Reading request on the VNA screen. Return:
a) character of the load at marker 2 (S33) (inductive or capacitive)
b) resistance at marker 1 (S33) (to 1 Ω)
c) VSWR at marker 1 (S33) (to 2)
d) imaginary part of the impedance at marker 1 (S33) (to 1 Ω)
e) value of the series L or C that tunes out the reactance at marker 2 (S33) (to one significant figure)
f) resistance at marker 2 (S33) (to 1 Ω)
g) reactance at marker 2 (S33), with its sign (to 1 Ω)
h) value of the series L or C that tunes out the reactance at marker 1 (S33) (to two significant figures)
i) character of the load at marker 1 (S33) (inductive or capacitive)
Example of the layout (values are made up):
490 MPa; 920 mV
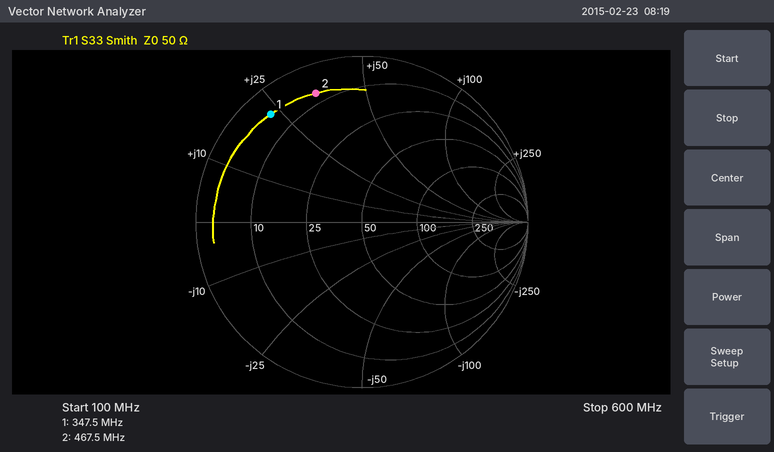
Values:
inductive; 5 Ω; 12; +23 Ω; 10 pF; 7 Ω; +35 Ω; 20 pF; inductive
